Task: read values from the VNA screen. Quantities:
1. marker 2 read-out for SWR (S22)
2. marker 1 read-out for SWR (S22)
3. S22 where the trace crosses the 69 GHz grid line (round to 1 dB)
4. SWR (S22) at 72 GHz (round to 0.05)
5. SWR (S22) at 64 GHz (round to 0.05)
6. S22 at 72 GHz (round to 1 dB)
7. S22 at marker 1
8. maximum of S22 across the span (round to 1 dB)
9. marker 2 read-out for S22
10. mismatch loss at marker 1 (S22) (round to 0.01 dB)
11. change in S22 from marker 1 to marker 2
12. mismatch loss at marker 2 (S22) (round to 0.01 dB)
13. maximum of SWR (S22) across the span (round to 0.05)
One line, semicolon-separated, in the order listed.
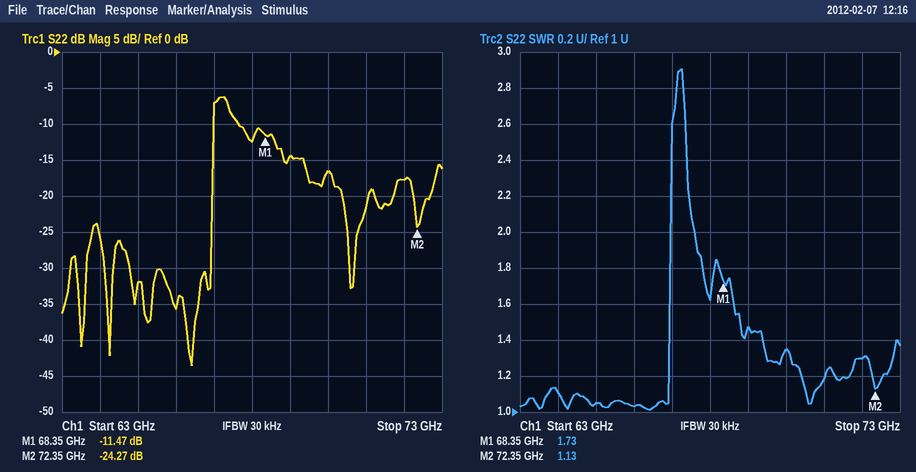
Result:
1.13; 1.73; -14 dB; 1.30; 1.10; -18 dB; -11.47 dB; -6 dB; -24.27 dB; 0.32 dB; -12.80 dB; 0.02 dB; 2.90
